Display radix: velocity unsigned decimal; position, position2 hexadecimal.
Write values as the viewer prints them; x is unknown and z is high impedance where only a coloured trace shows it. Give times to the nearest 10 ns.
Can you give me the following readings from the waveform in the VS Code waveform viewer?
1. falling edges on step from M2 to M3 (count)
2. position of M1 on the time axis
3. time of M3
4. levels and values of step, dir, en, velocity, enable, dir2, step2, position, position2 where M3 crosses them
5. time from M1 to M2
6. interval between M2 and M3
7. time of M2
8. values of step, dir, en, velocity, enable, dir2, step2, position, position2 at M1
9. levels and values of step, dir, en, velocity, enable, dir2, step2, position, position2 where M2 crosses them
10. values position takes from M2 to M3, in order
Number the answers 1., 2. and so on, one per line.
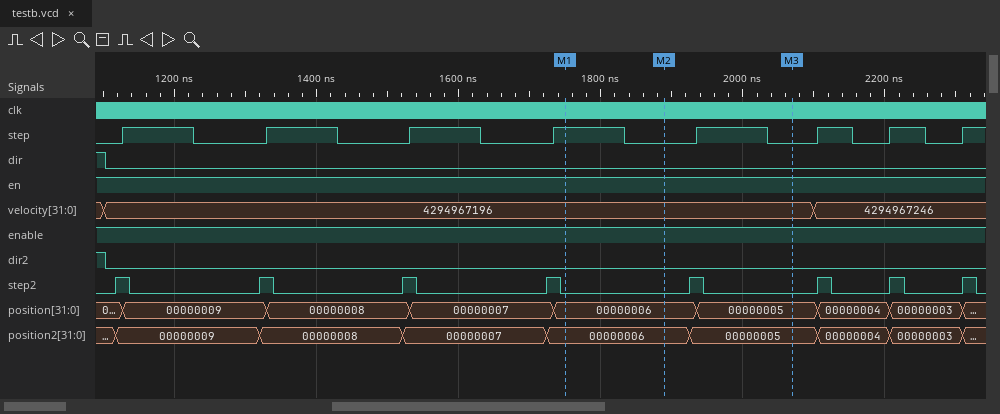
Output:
1. 1
2. 1750 ns
3. 2070 ns
4. step=0, dir=0, en=1, velocity=4294967196, enable=1, dir2=0, step2=0, position=00000005, position2=00000005
5. 140 ns
6. 180 ns
7. 1890 ns
8. step=1, dir=0, en=1, velocity=4294967196, enable=1, dir2=0, step2=0, position=00000006, position2=00000006
9. step=0, dir=0, en=1, velocity=4294967196, enable=1, dir2=0, step2=0, position=00000006, position2=00000006
10. 00000006, 00000005
